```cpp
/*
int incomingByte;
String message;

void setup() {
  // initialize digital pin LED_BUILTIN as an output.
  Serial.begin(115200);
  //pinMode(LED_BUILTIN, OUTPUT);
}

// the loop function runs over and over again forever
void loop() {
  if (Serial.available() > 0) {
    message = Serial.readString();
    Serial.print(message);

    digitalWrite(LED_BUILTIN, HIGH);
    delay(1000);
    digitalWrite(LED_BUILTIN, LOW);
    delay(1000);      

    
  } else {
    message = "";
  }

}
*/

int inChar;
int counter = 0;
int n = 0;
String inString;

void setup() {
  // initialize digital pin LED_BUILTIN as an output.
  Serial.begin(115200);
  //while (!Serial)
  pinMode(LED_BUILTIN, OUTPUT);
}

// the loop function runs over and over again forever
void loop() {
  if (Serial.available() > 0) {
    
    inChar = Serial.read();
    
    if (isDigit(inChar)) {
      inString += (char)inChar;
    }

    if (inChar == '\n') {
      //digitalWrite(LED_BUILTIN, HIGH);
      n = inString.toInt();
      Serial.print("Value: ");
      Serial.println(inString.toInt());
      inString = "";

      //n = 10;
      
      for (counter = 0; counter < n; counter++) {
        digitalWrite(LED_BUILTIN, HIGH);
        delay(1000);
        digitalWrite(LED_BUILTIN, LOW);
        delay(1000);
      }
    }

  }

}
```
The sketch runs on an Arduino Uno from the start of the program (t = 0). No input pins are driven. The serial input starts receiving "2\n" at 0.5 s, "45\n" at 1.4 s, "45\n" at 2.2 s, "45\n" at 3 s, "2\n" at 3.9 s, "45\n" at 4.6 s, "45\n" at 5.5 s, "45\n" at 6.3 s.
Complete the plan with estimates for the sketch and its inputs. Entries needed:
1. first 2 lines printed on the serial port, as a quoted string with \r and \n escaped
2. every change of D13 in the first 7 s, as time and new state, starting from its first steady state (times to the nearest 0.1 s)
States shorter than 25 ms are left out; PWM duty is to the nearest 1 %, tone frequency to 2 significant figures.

"Value: 2\r\nValue: 45\r\n"
0 s low; 0.5 s high; 1.5 s low; 2.5 s high; 3.5 s low; 4.5 s high; 5.5 s low; 6.5 s high
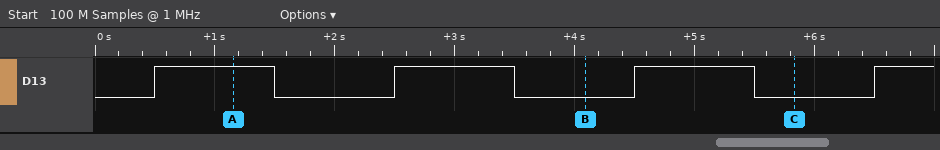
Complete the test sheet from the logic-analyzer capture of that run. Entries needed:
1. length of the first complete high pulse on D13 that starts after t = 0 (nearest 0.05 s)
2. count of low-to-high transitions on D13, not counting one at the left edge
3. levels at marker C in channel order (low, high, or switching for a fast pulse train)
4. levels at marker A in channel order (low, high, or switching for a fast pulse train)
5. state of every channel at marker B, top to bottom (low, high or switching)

1.00 s
4
D13 low
D13 high
D13 low
